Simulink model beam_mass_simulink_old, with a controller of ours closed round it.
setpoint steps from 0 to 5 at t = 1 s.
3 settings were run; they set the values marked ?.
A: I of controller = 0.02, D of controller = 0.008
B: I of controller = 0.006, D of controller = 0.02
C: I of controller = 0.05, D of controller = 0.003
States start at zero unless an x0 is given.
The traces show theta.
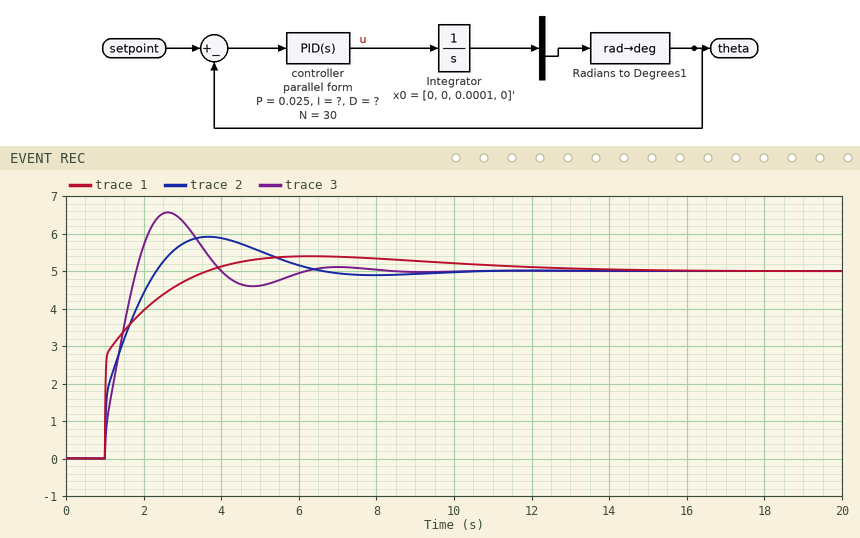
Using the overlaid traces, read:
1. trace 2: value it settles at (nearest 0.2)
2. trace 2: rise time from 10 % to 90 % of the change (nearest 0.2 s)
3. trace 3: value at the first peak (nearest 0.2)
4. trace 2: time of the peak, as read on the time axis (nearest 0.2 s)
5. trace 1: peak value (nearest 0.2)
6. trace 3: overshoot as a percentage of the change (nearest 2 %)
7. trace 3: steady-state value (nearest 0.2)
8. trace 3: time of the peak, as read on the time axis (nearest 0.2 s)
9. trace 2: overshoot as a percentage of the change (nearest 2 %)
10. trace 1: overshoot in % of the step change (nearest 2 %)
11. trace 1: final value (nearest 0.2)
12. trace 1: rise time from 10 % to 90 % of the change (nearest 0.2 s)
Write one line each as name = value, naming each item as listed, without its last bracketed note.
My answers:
trace 2: value it settles at = 5.0
trace 2: rise time from 10 % to 90 % of the change = 1.0 s
trace 3: value at the first peak = 6.6
trace 2: time of the peak, as read on the time axis = 3.6 s
trace 1: peak value = 5.4
trace 3: overshoot as a percentage of the change = 32 %
trace 3: steady-state value = 5.0
trace 3: time of the peak, as read on the time axis = 2.6 s
trace 2: overshoot as a percentage of the change = 18 %
trace 1: overshoot in % of the step change = 8 %
trace 1: final value = 5.0
trace 1: rise time from 10 % to 90 % of the change = 1.6 s
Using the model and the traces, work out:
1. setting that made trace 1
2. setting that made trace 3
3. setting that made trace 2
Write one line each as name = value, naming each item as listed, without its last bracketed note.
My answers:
setting that made trace 1 = B
setting that made trace 3 = C
setting that made trace 2 = A
